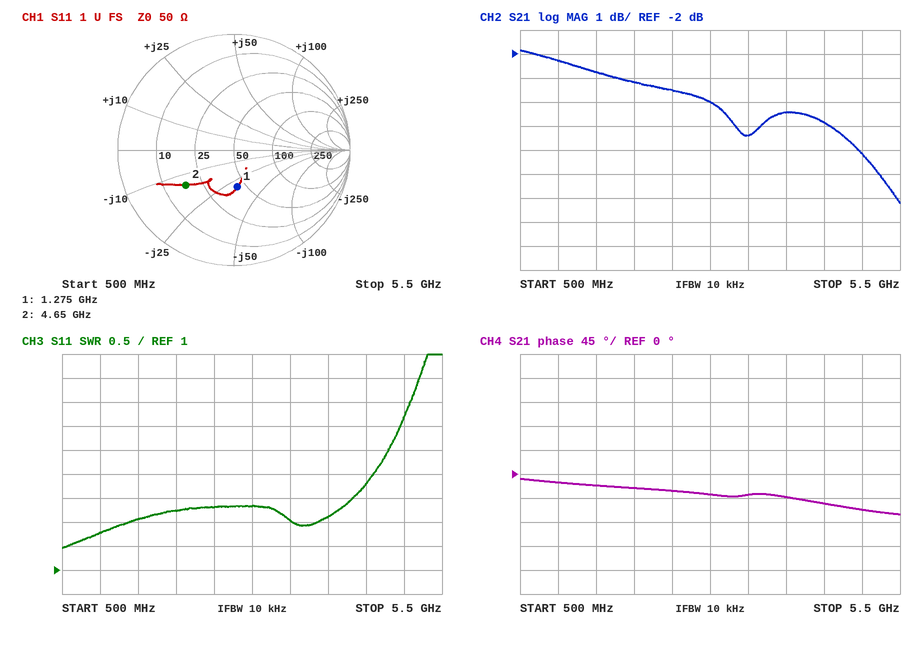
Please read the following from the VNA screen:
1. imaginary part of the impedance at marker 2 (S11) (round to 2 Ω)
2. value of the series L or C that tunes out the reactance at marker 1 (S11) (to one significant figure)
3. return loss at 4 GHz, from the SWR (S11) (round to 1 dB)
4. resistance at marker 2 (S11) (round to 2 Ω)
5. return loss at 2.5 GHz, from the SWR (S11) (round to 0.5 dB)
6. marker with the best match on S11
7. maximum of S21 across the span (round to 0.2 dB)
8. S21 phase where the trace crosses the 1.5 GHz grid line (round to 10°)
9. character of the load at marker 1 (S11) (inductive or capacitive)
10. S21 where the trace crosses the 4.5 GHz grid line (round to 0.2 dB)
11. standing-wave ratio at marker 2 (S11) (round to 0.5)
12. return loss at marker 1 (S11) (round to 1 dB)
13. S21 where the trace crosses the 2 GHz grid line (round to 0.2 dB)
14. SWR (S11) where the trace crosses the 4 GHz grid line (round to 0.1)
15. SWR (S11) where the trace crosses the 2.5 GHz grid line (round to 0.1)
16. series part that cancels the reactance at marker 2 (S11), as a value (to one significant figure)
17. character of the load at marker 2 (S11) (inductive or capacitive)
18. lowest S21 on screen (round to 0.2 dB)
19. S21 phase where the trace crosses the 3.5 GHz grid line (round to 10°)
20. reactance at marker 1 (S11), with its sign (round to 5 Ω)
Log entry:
-14 Ω
4 nH
9 dB
18 Ω
8.0 dB
marker 1
-1.8 dB
-20°
capacitive
-4.8 dB
3.0
10 dB
-3.2 dB
2.1
2.3
500 pH
capacitive
-8.2 dB
-40°
-30 Ω
